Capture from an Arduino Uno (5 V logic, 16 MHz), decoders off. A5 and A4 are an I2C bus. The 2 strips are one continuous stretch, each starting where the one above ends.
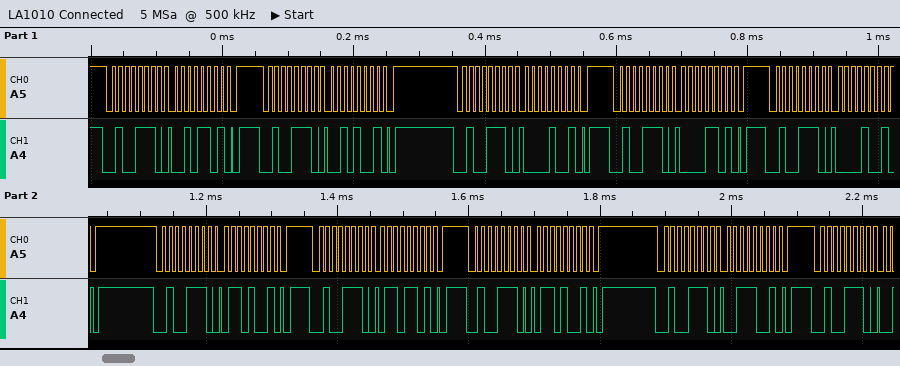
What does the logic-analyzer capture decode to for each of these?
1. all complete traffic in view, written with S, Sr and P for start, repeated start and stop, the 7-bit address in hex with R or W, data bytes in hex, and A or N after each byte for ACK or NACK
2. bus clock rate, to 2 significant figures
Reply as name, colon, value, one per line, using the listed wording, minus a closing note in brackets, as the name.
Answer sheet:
all complete traffic in view, written with S, Sr and P for start, repeated start and stop, the 7-bit address in hex with R or W, data bytes in hex, and A or N after each byte for ACK or NACK: S 27W A 2D A P S 27W A 29 A P S 27W A 09 A P S 27W A 0D A P S 27W A 09 A P S 27W A 69 A P S 27W A 6D A P S 27W A 69 A P S 27W A 39 A P S 27W A
bus clock rate, to 2 significant figures: 100 kHz
